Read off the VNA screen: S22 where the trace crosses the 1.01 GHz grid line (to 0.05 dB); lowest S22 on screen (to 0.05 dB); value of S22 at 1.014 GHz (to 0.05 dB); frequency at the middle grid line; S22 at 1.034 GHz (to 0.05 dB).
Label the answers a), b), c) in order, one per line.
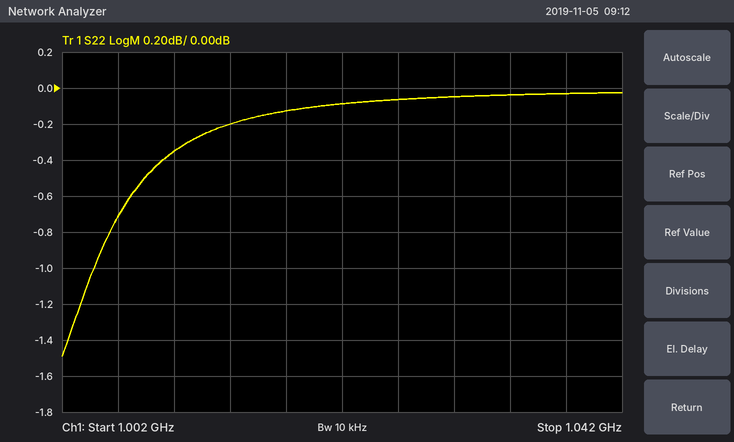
a) -0.35 dB
b) -1.50 dB
c) -0.20 dB
d) 1.022 GHz
e) -0.05 dB
